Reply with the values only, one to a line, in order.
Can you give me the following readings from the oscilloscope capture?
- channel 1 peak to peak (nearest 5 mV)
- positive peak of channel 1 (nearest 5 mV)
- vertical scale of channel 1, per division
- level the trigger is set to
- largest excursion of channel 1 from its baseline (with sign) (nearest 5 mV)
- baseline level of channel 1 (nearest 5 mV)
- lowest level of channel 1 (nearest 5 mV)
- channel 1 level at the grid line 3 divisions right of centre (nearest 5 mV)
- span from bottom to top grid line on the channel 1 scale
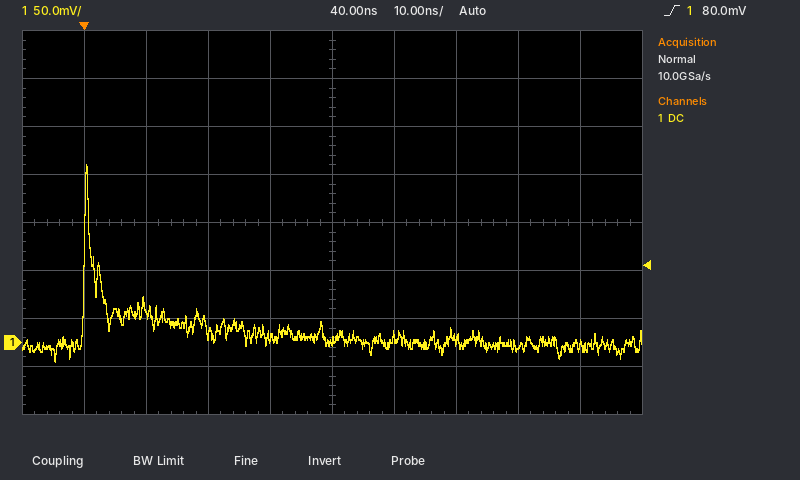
205 mV
185 mV
50 mV
80.0 mV
+185 mV
0 mV
-20 mV
-5 mV
400 mV
